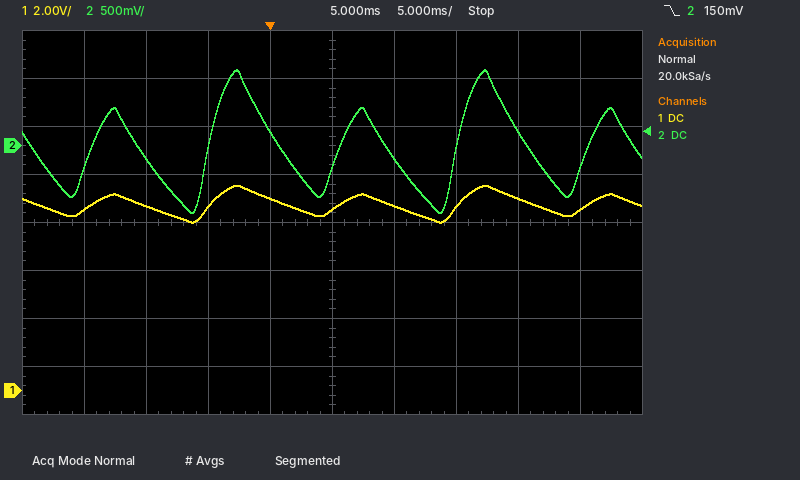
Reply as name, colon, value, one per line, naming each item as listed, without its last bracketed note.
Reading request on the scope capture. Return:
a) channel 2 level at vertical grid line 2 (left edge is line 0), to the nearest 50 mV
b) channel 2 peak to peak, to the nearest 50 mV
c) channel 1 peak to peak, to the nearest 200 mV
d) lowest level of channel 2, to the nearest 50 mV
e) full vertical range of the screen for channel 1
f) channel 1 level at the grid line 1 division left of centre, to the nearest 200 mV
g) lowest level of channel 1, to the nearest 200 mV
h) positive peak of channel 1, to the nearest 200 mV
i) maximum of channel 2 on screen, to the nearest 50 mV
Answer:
channel 2 level at vertical grid line 2 (left edge is line 0), to the nearest 50 mV: -150 mV
channel 2 peak to peak, to the nearest 50 mV: 1.50 V
channel 1 peak to peak, to the nearest 200 mV: 1.6 V
lowest level of channel 2, to the nearest 50 mV: -700 mV
full vertical range of the screen for channel 1: 16 V
channel 1 level at the grid line 1 division left of centre, to the nearest 200 mV: 8.0 V
lowest level of channel 1, to the nearest 200 mV: 7.0 V
positive peak of channel 1, to the nearest 200 mV: 8.6 V
maximum of channel 2 on screen, to the nearest 50 mV: 800 mV
